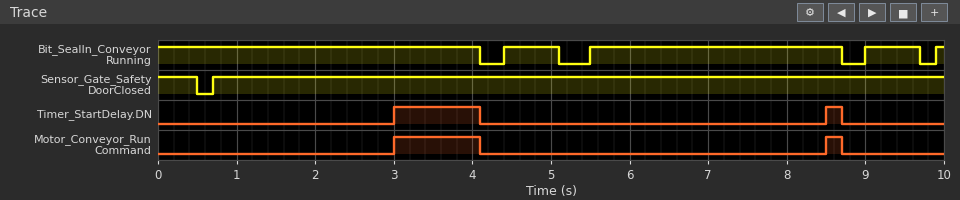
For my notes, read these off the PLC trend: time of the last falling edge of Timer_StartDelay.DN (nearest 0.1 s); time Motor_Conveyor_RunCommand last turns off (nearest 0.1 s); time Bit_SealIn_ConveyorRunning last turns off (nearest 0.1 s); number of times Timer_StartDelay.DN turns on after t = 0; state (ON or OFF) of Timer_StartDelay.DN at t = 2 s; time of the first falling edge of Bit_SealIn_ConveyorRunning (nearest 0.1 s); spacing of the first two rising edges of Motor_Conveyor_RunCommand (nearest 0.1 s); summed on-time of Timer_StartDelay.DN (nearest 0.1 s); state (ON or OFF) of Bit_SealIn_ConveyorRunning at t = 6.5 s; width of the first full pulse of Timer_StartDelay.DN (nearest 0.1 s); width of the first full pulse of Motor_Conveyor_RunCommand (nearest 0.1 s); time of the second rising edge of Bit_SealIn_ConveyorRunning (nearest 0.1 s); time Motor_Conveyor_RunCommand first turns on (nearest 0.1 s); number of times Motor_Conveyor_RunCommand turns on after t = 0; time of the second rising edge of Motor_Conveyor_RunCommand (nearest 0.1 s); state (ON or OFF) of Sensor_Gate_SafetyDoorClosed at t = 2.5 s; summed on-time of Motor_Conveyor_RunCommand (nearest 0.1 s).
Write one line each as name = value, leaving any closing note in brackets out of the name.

time of the last falling edge of Timer_StartDelay.DN = 8.7 s
time Motor_Conveyor_RunCommand last turns off = 8.7 s
time Bit_SealIn_ConveyorRunning last turns off = 9.7 s
number of times Timer_StartDelay.DN turns on after t = 0 = 2
state (ON or OFF) of Timer_StartDelay.DN at t = 2 s = OFF
time of the first falling edge of Bit_SealIn_ConveyorRunning = 4.1 s
spacing of the first two rising edges of Motor_Conveyor_RunCommand = 5.5 s
summed on-time of Timer_StartDelay.DN = 1.3 s
state (ON or OFF) of Bit_SealIn_ConveyorRunning at t = 6.5 s = ON
width of the first full pulse of Timer_StartDelay.DN = 1.1 s
width of the first full pulse of Motor_Conveyor_RunCommand = 1.1 s
time of the second rising edge of Bit_SealIn_ConveyorRunning = 5.5 s
time Motor_Conveyor_RunCommand first turns on = 3.0 s
number of times Motor_Conveyor_RunCommand turns on after t = 0 = 2
time of the second rising edge of Motor_Conveyor_RunCommand = 8.5 s
state (ON or OFF) of Sensor_Gate_SafetyDoorClosed at t = 2.5 s = ON
summed on-time of Motor_Conveyor_RunCommand = 1.3 s
